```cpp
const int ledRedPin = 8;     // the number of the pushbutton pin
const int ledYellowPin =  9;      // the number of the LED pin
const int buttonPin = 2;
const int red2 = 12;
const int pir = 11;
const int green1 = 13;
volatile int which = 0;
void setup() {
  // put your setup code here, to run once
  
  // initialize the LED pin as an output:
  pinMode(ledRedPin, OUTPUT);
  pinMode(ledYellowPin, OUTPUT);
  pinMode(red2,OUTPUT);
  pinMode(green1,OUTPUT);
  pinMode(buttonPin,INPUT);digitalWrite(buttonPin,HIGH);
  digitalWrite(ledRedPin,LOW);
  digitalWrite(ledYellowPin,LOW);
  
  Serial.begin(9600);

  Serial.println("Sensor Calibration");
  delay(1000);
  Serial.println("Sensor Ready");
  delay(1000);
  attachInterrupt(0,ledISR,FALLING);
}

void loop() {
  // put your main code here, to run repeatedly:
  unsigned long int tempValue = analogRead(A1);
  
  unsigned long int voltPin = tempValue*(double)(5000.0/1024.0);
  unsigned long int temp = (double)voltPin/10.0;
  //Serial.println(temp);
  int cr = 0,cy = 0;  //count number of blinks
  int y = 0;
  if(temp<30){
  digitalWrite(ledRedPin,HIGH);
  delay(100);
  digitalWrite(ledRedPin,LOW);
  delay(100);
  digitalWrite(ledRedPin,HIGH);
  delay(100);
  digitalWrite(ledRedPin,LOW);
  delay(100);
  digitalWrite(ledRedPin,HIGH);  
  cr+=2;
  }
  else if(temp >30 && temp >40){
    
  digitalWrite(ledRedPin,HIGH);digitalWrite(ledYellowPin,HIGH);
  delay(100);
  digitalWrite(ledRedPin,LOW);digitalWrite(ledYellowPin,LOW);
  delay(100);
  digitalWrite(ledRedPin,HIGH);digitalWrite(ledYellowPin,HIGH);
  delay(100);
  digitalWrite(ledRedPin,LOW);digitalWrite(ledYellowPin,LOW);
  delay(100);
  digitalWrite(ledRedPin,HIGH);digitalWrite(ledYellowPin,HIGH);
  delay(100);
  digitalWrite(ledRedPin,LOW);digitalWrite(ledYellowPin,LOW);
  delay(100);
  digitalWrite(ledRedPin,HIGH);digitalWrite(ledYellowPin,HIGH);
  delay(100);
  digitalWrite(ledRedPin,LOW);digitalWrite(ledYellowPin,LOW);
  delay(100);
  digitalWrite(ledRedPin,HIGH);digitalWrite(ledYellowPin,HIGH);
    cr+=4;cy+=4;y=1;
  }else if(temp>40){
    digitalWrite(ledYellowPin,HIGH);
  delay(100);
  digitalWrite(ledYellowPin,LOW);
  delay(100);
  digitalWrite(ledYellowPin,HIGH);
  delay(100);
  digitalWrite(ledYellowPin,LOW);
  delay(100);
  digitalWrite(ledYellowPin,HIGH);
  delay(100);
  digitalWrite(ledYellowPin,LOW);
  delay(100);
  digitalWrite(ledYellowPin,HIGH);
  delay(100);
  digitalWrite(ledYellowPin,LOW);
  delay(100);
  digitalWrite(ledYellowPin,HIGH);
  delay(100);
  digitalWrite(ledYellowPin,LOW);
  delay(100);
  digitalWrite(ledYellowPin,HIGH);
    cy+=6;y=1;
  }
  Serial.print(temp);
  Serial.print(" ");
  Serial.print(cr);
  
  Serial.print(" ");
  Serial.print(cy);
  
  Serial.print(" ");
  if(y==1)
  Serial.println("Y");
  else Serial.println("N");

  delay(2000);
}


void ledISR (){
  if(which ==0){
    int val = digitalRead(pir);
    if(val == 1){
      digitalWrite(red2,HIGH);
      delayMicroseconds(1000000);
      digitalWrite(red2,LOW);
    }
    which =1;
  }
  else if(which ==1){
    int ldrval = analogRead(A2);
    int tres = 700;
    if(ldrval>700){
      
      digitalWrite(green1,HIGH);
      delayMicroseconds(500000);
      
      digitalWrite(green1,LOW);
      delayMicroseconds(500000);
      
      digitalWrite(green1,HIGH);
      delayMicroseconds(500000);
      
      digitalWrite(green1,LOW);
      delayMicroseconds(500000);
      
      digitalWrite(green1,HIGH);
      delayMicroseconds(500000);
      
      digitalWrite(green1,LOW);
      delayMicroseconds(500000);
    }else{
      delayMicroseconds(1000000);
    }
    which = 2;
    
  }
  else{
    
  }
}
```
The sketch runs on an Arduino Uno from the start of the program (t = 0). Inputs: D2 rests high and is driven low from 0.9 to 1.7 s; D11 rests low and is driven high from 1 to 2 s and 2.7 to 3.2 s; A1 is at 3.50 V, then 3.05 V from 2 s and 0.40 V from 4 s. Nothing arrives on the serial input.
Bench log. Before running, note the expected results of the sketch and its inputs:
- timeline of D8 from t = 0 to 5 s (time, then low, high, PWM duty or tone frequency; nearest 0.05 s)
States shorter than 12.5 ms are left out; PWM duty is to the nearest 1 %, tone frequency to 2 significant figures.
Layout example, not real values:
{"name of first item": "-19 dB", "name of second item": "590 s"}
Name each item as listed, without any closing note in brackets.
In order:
{"timeline of D8 from t = 0 to 5 s": "0 s low; 2 s high; 2.1 s low; 2.2 s high; 2.3 s low; 2.4 s high; 2.5 s low; 2.6 s high; 2.7 s low; 2.8 s high"}
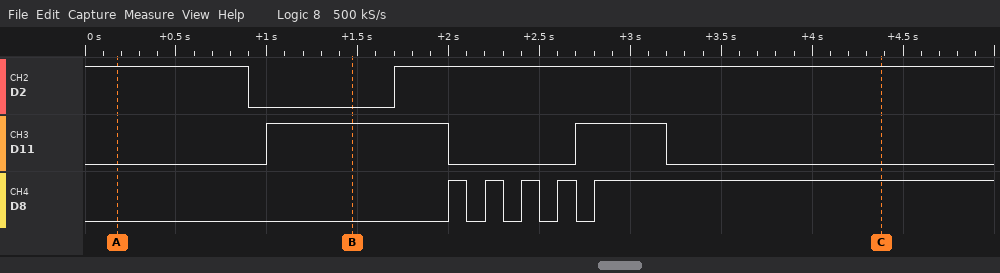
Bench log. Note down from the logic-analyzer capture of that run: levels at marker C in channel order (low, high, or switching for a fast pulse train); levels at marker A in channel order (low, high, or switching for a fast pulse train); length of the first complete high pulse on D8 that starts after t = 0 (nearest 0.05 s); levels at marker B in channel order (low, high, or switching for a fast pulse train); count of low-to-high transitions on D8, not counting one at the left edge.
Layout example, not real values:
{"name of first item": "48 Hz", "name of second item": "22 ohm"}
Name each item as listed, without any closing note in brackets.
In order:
{"levels at marker C in channel order": "D2 high, D11 low, D8 high", "levels at marker A in channel order": "D2 high, D11 low, D8 low", "length of the first complete high pulse on D8 that starts after t = 0": "0.10 s", "levels at marker B in channel order": "D2 low, D11 high, D8 low", "count of low-to-high transitions on D8, not counting one at the left edge": "5"}
